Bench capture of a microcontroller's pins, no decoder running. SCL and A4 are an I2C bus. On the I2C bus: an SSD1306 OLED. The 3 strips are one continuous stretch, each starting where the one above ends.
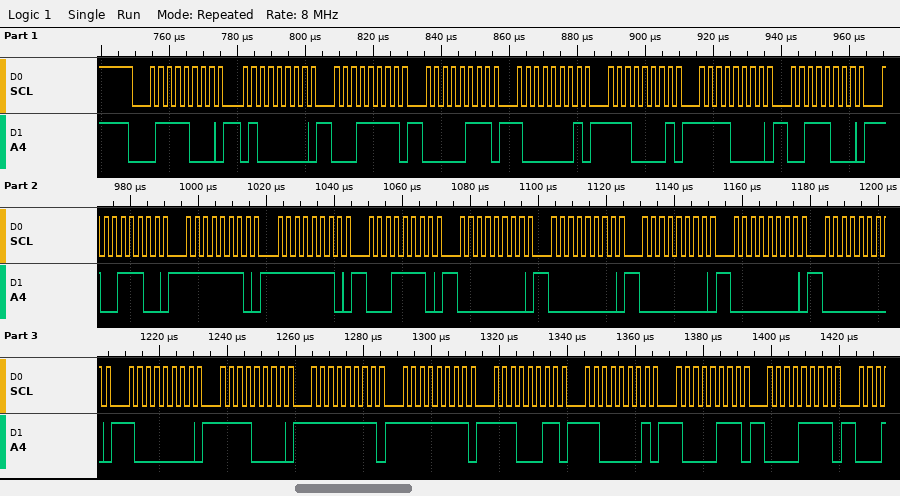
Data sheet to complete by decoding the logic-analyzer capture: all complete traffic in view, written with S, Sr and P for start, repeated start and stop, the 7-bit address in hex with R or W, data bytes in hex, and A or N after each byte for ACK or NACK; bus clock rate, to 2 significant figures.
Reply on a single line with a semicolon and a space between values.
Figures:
S 3CW A 40 A 1F A 07 A 81 A E1 A F0 A 38 A 9C A FE A FE A 1E A 00 A 00 A 00 A 00 A 00 A 80 A F0 A FF A FF A E3 A C1 A 87 A 0F A; 400 kHz
